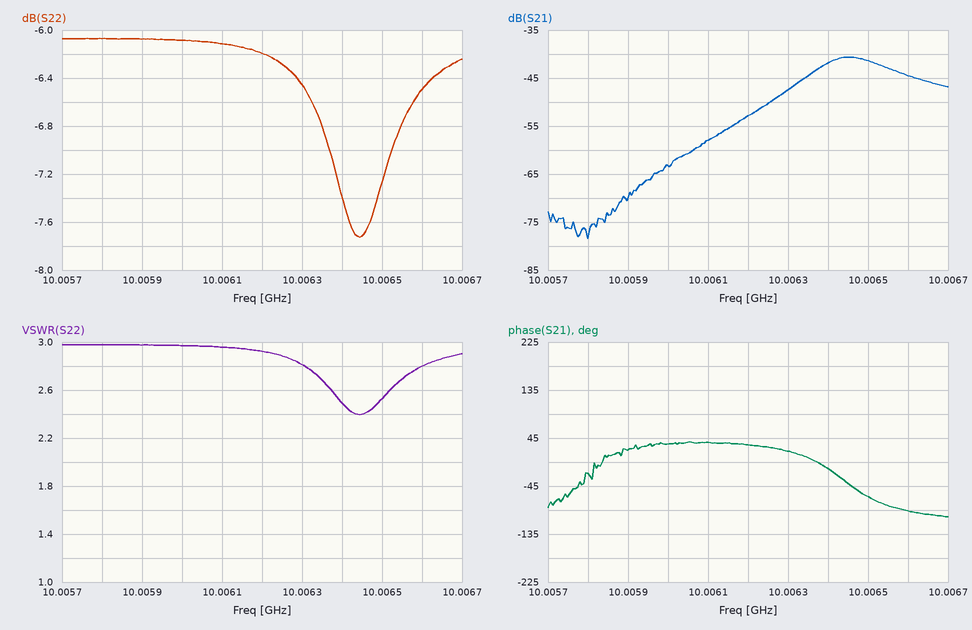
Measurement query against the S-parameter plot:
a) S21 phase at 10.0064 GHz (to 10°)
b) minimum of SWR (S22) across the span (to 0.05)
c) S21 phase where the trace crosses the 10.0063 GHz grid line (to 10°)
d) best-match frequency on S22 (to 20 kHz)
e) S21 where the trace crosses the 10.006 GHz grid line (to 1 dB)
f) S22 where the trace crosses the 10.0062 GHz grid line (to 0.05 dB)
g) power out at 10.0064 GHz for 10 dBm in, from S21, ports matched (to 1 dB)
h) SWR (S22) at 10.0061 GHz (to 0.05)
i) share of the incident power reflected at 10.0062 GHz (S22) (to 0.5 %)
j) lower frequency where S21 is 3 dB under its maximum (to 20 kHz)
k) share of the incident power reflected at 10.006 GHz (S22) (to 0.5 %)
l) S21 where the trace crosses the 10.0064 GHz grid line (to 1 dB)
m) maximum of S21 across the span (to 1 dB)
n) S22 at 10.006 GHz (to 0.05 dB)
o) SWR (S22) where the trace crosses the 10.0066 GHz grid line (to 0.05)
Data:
-10°
2.40
20°
10.00644 GHz
-63 dB
-6.20 dB
-32 dBm
2.95
24.0 %
10.00636 GHz
24.5 %
-42 dB
-41 dB
-6.10 dB
2.80
